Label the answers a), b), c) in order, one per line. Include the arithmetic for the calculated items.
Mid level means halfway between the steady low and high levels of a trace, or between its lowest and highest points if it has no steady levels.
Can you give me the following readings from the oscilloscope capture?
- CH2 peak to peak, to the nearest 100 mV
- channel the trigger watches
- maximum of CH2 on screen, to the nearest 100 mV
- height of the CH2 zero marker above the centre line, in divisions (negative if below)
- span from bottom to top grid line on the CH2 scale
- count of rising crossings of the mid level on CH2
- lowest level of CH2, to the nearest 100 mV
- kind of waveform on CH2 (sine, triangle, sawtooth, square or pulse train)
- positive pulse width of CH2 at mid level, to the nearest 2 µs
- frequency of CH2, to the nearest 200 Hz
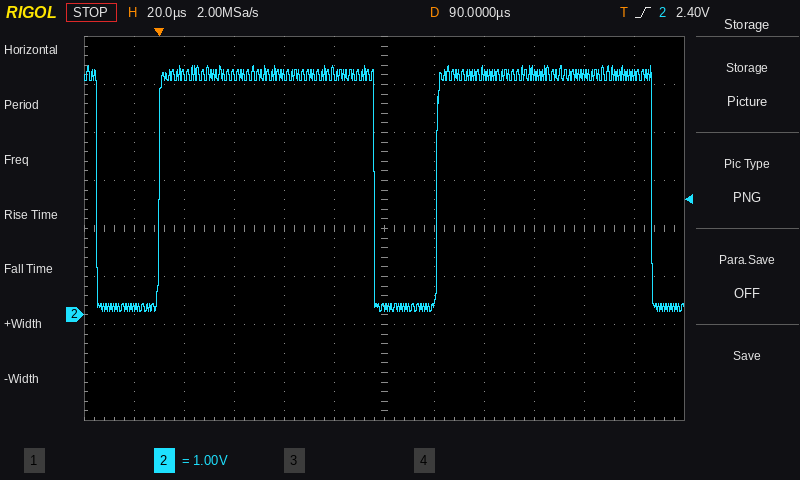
a) 5.2 V − (100 mV) = 5.1 V
b) CH2
c) 5.2 V
d) -1.8 div
e) 8 V
f) 2
g) 100 mV
h) pulse train
i) 86 µs
j) 9.0 kHz
